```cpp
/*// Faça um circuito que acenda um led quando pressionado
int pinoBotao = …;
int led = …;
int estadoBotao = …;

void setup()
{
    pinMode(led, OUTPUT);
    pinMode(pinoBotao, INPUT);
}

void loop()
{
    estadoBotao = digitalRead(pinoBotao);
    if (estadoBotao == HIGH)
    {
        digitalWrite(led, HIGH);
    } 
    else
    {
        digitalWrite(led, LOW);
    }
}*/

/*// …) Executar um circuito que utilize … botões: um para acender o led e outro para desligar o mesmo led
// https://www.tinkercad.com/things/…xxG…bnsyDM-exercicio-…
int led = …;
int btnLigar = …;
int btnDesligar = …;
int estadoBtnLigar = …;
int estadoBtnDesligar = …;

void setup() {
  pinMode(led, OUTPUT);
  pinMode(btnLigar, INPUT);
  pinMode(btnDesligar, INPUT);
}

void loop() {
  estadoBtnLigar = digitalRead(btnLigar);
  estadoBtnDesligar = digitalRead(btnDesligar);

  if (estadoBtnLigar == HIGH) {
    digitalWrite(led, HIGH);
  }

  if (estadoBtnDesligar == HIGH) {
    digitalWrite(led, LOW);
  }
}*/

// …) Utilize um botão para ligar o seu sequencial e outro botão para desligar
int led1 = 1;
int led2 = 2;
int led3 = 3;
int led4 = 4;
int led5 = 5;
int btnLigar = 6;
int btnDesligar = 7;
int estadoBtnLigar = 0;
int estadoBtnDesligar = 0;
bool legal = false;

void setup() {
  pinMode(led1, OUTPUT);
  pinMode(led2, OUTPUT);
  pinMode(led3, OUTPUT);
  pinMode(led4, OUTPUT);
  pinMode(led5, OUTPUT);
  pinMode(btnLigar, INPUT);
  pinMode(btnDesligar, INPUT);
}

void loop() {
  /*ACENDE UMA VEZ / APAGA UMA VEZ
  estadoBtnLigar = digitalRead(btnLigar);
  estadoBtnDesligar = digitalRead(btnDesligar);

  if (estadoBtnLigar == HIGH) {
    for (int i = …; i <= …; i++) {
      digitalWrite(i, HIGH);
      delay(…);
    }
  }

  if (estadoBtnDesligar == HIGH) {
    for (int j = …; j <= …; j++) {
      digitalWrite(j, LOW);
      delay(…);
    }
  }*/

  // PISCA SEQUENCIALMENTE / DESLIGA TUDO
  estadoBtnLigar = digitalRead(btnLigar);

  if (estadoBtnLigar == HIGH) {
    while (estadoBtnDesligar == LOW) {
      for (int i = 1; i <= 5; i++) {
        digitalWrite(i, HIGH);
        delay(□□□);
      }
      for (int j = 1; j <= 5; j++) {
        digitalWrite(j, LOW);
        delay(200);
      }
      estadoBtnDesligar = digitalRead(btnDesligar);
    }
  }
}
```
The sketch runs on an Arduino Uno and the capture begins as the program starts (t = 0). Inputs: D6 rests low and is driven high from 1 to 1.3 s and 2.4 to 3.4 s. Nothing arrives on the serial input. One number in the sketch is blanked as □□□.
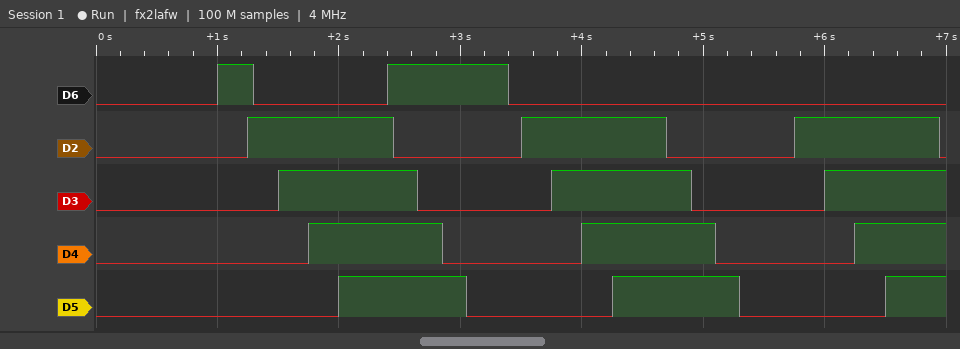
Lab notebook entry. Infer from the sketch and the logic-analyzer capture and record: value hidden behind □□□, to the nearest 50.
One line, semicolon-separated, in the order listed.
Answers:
250
